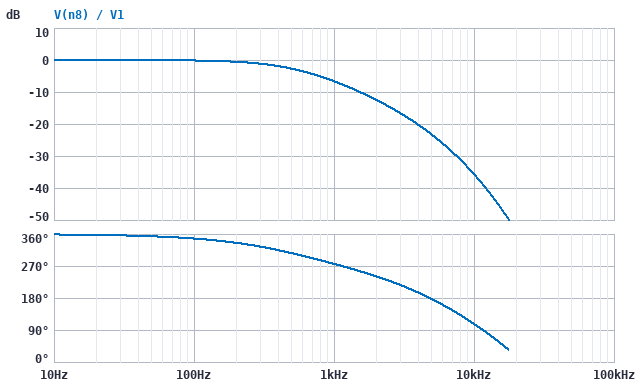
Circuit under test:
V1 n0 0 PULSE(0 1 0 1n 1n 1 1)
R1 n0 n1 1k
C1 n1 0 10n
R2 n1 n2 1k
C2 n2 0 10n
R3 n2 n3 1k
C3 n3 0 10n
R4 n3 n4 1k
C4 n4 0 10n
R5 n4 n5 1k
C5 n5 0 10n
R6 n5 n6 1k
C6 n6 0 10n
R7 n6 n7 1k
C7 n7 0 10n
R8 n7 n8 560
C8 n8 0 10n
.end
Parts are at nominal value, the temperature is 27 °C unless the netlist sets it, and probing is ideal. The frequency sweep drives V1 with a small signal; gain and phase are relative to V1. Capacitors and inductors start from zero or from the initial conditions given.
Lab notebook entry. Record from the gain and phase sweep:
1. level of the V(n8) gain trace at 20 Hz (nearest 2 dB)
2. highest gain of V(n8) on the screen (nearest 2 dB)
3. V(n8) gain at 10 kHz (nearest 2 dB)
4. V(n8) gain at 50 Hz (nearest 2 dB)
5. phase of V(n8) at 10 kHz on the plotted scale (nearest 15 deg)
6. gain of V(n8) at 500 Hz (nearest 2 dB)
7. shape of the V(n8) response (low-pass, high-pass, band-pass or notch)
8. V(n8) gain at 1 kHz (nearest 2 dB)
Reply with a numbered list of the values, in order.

1. 0 dB
2. 0 dB
3. -36 dB
4. 0 dB
5. 105 deg
6. -2 dB
7. low-pass
8. -6 dB
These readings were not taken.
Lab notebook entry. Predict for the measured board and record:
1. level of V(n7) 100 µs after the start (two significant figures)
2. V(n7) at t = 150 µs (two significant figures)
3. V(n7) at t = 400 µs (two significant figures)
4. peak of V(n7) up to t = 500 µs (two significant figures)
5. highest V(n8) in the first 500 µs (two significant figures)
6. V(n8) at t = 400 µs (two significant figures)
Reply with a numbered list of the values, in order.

1. 140 mV
2. 270 mV
3. 690 mV
4. 780 mV
5. 770 mV
6. 680 mV
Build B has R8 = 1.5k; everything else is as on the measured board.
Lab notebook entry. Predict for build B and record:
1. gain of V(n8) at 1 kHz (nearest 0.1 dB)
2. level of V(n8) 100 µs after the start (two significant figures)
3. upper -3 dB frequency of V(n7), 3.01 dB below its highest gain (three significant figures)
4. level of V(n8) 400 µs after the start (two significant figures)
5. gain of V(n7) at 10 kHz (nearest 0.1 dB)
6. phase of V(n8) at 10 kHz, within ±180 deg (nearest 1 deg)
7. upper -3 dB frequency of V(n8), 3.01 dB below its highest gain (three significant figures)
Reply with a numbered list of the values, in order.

1. -6.7 dB
2. 110 mV
3. 532 Hz
4. 670 mV
5. -34.4 dB
6. 91 deg
7. 531 Hz
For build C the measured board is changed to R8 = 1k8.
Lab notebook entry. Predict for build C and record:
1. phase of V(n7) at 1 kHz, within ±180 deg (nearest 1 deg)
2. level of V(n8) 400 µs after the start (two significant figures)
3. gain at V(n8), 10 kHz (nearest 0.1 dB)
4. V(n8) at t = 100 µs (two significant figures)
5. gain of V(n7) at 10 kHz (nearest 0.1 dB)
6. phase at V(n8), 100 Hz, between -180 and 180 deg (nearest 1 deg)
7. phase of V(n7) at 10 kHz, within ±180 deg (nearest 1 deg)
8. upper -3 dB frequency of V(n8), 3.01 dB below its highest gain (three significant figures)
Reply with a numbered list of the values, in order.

1. -81 deg
2. 670 mV
3. -37.7 dB
4. 110 mV
5. -34.1 dB
6. -13 deg
7. 136 deg
8. 529 Hz
